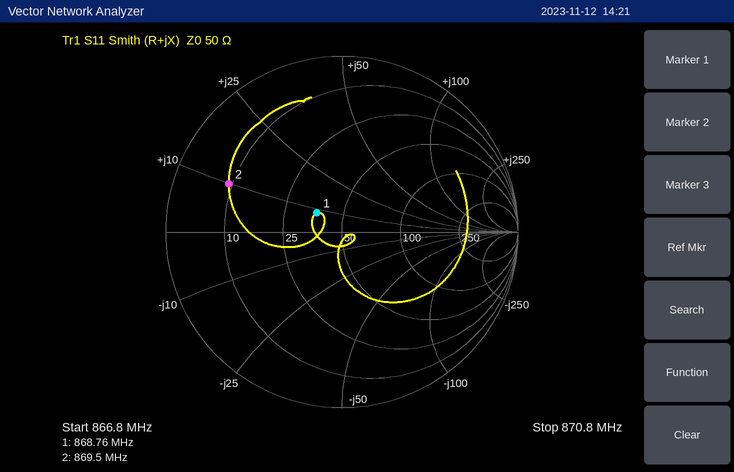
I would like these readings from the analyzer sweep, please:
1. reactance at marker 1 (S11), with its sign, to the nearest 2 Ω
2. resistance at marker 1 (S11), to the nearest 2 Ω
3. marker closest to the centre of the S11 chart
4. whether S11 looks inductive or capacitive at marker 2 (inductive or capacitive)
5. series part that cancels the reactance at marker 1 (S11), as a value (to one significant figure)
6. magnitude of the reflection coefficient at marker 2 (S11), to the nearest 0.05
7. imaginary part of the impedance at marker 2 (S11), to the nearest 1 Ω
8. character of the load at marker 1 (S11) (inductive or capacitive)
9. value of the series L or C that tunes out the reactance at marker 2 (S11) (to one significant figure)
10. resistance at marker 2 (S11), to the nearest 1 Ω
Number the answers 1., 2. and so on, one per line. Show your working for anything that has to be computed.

1. +8 Ω
2. 36 Ω
3. marker 1
4. inductive
5. C = 1/(2π × 868.76 MHz × 8 Ω) ≈ 22.9 pF, so 20 pF to one significant figure
6. 0.70
7. +10 Ω
8. inductive
9. C = 1/(2π × 869.5 MHz × 10 Ω) ≈ 18.3 pF, so 20 pF to one significant figure
10. 9 Ω
